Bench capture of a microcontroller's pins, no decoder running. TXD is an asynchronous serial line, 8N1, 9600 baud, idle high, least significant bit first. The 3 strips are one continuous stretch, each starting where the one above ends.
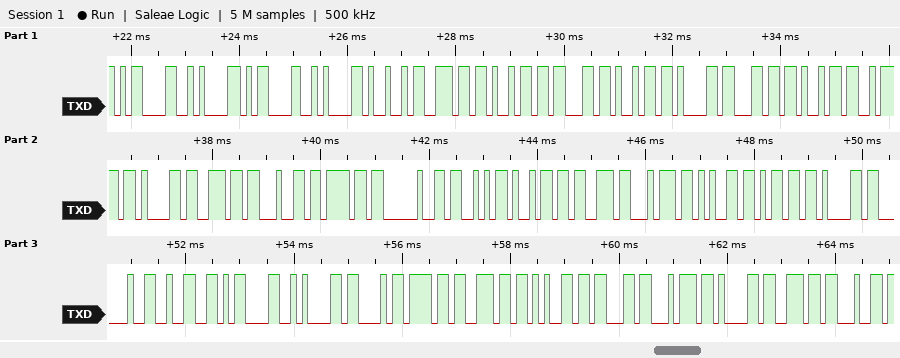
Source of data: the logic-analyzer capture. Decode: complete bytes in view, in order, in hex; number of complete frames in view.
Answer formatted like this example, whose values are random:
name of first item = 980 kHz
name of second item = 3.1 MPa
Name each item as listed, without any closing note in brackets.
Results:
complete bytes in view, in order, in hex = 0D 0A 0D 0A 49 6E 69 63 69 61 6C 69 7A 61 6E 64 6F 20 53 69 73 74 65 6D 61 20 32 0D 0A 43 6F 6E 65 63 74 61 6E 64
number of complete frames in view = 38
